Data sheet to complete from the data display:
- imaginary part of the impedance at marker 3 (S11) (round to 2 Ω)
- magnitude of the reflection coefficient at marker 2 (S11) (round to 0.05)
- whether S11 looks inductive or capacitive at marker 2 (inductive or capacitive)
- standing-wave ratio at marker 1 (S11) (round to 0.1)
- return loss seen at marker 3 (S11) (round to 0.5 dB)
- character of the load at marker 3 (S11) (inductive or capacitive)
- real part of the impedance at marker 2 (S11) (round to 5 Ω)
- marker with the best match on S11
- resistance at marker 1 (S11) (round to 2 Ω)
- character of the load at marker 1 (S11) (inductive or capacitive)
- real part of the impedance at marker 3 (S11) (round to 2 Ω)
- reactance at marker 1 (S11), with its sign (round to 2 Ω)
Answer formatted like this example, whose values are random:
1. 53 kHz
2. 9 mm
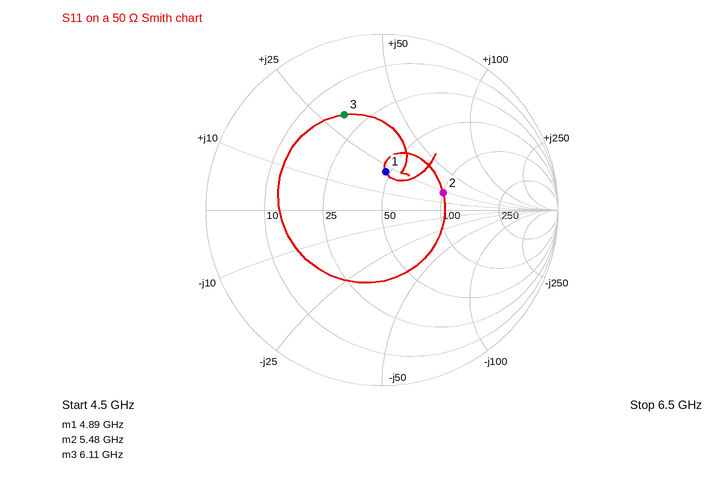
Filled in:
1. +30 Ω
2. 0.35
3. inductive
4. 1.6
5. 4.5 dB
6. inductive
7. 100 Ω
8. marker 1
9. 48 Ω
10. inductive
11. 18 Ω
12. +22 Ω
